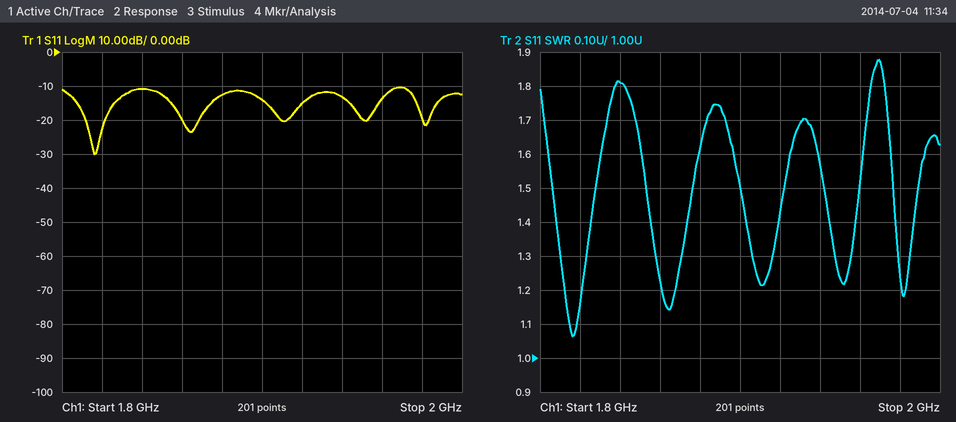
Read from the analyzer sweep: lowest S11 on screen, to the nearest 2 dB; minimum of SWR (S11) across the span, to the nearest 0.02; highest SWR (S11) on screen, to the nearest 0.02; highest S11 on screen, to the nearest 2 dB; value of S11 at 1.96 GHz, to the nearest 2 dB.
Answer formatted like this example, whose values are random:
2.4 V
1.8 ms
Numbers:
-30 dB
1.06
1.88
-10 dB
-14 dB
